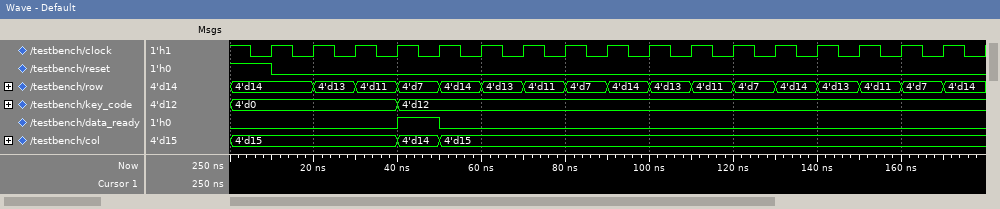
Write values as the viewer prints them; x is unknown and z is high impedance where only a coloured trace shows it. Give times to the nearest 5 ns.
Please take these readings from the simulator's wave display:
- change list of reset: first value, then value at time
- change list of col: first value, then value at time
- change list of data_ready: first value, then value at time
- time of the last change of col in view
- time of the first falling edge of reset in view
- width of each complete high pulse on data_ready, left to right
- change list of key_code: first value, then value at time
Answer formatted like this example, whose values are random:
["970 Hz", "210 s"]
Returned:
["1, 0 at 10 ns", "4'd15, 4'd14 at 40 ns, 4'd15 at 50 ns", "0, 1 at 40 ns, 0 at 50 ns", "50 ns", "10 ns", "10 ns", "4'd0, 4'd12 at 40 ns"]
